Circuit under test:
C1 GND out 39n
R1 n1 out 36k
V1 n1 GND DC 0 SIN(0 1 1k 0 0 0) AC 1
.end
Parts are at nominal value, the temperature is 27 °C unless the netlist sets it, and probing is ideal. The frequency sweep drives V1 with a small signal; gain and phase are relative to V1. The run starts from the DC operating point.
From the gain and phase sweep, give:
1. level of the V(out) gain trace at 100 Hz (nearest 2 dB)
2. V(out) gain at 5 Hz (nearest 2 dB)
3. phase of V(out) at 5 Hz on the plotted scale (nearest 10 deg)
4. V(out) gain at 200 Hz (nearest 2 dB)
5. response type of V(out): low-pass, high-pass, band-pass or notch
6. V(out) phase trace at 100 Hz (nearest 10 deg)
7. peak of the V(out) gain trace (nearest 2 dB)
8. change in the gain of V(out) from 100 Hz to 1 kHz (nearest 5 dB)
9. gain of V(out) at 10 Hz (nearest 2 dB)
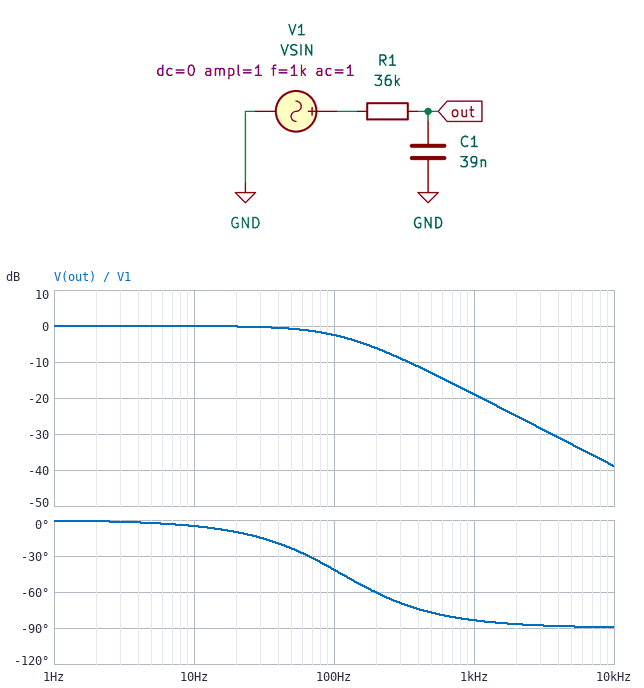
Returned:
-2 dB
0 dB
0 deg
-6 dB
low-pass
-40 deg
0 dB
-15 dB
0 dB
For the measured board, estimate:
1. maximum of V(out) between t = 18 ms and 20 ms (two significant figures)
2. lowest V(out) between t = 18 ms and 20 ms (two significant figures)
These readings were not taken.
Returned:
110 mV
-110 mV
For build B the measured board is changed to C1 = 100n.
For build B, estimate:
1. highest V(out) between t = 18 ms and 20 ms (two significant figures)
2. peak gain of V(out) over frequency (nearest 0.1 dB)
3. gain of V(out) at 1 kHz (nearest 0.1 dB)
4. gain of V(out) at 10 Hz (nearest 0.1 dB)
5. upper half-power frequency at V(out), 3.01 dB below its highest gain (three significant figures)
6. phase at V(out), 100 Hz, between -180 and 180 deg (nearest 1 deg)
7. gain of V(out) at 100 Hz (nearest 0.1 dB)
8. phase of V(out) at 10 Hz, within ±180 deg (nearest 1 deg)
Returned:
44 mV
0 dB
-27.1 dB
-0.2 dB
44.2 Hz
-66 deg
-7.9 dB
-13 deg
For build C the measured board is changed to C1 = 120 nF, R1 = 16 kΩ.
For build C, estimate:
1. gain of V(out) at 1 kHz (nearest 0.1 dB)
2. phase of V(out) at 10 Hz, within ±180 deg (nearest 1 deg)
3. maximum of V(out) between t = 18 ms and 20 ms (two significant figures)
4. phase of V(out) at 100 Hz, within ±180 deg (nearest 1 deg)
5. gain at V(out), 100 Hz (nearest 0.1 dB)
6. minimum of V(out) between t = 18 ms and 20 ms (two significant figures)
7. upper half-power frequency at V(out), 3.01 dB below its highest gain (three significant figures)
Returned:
-21.7 dB
-7 deg
83 mV
-50 deg
-3.9 dB
-83 mV
82.9 Hz
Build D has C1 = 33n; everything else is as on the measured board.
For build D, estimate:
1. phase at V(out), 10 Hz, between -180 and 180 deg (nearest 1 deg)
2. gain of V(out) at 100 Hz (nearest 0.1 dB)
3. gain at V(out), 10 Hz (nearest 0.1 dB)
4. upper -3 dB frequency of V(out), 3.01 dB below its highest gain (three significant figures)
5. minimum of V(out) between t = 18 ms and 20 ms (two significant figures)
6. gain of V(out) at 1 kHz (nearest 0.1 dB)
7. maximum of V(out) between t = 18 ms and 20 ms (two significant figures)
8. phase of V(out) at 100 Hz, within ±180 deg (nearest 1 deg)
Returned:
-4 deg
-1.9 dB
0 dB
134 Hz
-130 mV
-17.5 dB
130 mV
-37 deg
